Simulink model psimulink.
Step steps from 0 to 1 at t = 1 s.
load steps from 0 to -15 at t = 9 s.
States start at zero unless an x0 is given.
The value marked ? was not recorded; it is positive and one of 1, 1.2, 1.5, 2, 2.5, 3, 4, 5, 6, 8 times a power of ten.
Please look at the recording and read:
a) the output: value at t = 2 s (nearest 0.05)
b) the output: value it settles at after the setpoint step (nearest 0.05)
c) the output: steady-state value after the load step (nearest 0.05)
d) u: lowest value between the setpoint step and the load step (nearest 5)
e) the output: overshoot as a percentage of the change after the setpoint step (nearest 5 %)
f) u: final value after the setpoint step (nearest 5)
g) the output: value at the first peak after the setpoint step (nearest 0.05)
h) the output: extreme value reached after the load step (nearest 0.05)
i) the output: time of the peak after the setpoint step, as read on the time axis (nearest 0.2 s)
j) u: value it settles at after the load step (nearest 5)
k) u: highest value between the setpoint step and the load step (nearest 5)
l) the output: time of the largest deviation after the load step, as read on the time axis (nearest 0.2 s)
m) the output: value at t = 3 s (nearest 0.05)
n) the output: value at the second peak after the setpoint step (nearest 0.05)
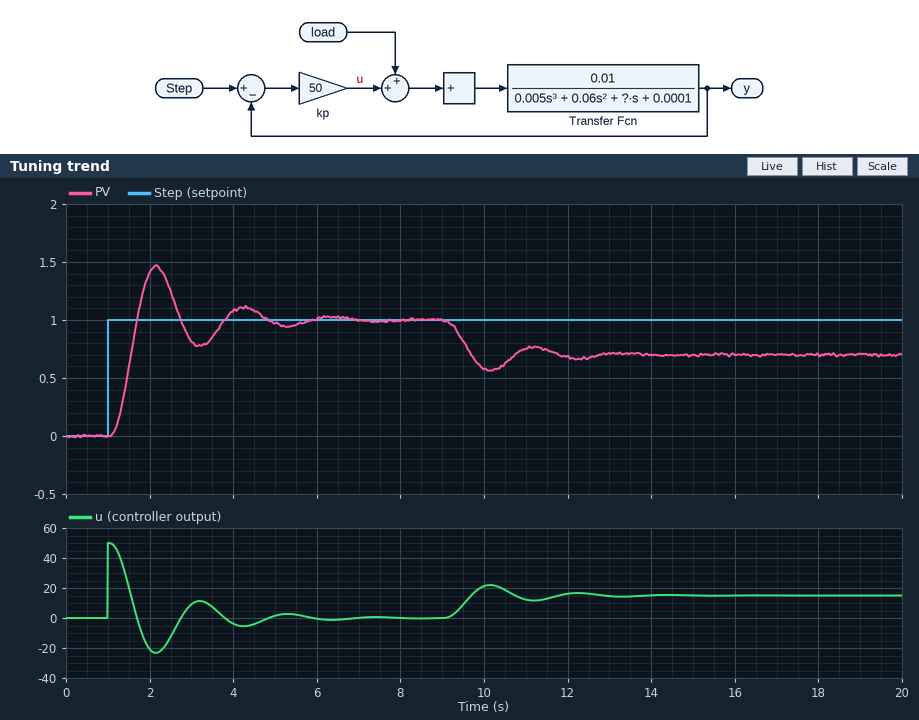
1.40
1.00
0.70
-25
45 %
0
1.45
0.55
2.2 s
15
50
10.2 s
0.80
1.10
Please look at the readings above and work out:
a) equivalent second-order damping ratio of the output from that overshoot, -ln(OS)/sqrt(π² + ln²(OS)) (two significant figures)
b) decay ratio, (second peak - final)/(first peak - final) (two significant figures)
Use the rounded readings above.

0.25
0.22
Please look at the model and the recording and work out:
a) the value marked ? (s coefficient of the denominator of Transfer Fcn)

0.12
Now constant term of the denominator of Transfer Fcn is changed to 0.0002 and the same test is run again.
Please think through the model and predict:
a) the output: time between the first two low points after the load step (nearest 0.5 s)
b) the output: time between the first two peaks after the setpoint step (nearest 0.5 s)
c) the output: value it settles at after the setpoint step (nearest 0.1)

2.0 s
2.0 s
1.0
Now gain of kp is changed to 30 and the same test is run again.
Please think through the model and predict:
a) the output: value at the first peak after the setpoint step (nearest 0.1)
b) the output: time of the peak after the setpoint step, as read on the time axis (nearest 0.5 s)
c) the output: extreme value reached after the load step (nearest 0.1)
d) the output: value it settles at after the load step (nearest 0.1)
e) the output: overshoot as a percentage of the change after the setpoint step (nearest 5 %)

1.3
2.5 s
0.4
0.5
30 %
